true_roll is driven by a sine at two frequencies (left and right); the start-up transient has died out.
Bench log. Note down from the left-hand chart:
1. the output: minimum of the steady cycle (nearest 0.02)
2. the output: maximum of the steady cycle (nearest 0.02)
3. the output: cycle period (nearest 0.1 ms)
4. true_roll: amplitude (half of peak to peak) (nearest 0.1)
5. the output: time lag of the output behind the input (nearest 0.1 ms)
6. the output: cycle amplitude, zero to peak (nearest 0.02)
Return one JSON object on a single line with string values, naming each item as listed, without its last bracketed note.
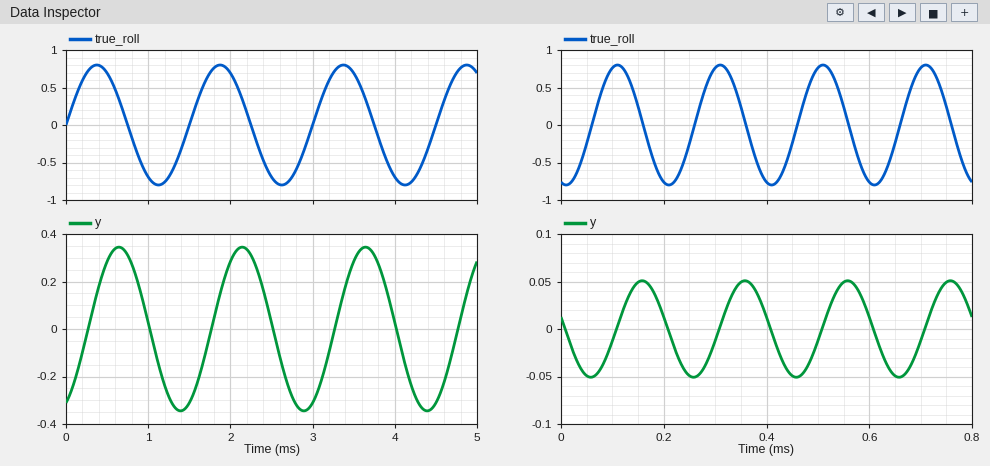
{"the output: minimum of the steady cycle": "-0.34", "the output: maximum of the steady cycle": "0.34", "the output: cycle period": "1.5 ms", "true_roll: amplitude (half of peak to peak)": "0.8", "the output: time lag of the output behind the input": "0.3 ms", "the output: cycle amplitude, zero to peak": "0.34"}
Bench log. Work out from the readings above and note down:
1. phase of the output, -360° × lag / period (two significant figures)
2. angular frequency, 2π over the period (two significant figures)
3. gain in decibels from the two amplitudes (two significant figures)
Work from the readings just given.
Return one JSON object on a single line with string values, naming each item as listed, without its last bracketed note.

{"phase of the output, -360° × lag / period": "-72°", "angular frequency, 2π over the period": "4.2 rad/ms", "gain in decibels from the two amplitudes": "-7.4 dB"}
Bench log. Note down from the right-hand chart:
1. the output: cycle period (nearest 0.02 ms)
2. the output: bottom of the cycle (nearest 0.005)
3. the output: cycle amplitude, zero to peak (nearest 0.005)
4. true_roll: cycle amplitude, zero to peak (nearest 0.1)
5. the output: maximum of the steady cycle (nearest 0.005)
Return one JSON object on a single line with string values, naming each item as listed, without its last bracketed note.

{"the output: cycle period": "0.20 ms", "the output: bottom of the cycle": "-0.050", "the output: cycle amplitude, zero to peak": "0.050", "true_roll: cycle amplitude, zero to peak": "0.8", "the output: maximum of the steady cycle": "0.050"}
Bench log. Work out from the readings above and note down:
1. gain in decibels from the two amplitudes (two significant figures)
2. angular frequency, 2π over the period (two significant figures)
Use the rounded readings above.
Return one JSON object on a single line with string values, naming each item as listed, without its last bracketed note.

{"gain in decibels from the two amplitudes": "-24 dB", "angular frequency, 2π over the period": "31 rad/ms"}
